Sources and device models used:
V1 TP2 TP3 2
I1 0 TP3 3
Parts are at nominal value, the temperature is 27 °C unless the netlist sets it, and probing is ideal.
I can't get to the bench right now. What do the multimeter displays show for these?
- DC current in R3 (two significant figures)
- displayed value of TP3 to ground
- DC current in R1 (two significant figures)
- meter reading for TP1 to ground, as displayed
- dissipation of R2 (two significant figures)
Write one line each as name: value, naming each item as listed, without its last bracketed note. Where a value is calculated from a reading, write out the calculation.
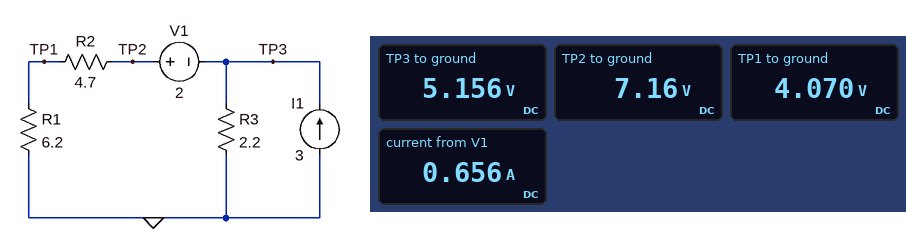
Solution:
DC current in R3: (5.156 V) / 2.2 Ω = 2.3 A
displayed value of TP3 to ground: 5.156 V
DC current in R1: (4.07 V) / 6.2 Ω = 660 mA
meter reading for TP1 to ground, as displayed: 4.070 V
dissipation of R2: (7.16 V - 4.07 V)^2 / 4.7 Ω = 2.0 W
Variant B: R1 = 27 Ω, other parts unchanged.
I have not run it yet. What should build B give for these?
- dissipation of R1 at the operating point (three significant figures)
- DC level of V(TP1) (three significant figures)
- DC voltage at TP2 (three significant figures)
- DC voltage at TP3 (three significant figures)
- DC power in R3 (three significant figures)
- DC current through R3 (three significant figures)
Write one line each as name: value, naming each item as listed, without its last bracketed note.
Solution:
dissipation of R1 at the operating point: 1.74 W
DC level of V(TP1): 6.85 V
DC voltage at TP2: 8.04 V
DC voltage at TP3: 6.04 V
DC power in R3: 16.6 W
DC current through R3: 2.75 A
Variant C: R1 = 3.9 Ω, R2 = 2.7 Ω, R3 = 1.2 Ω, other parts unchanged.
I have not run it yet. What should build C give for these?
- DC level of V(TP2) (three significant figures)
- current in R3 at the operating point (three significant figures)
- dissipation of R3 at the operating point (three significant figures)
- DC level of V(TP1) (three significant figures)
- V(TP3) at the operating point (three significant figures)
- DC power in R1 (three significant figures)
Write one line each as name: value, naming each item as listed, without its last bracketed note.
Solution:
DC level of V(TP2): 4.74 V
current in R3 at the operating point: 2.28 A
dissipation of R3 at the operating point: 6.25 W
DC level of V(TP1): 2.80 V
V(TP3) at the operating point: 2.74 V
DC power in R1: 2.01 W
